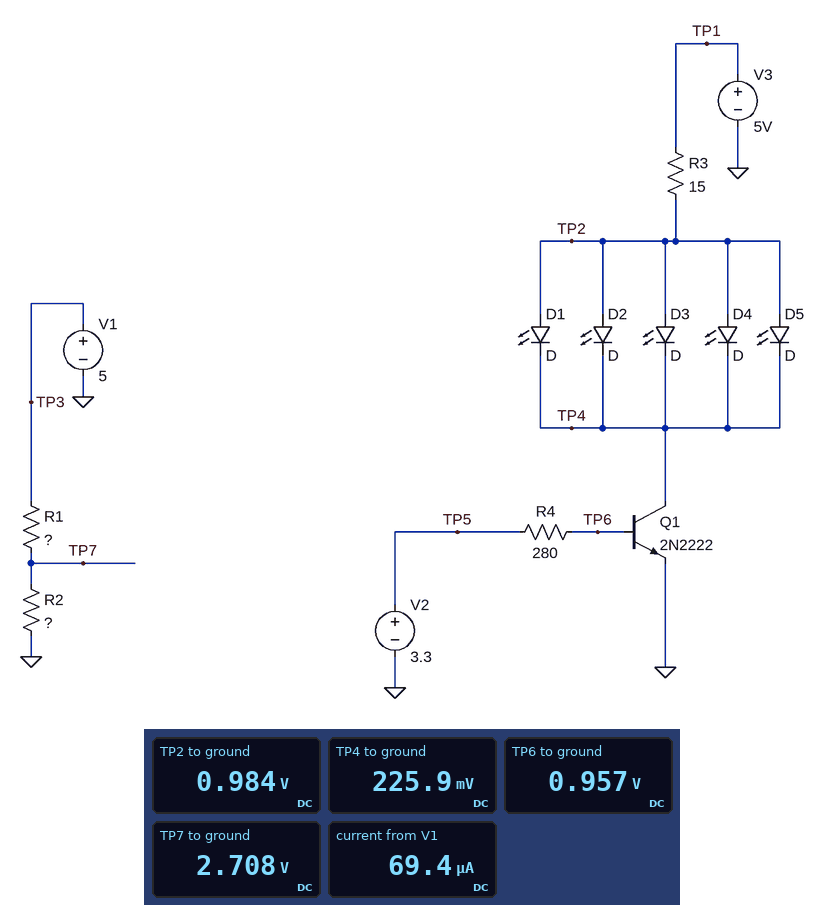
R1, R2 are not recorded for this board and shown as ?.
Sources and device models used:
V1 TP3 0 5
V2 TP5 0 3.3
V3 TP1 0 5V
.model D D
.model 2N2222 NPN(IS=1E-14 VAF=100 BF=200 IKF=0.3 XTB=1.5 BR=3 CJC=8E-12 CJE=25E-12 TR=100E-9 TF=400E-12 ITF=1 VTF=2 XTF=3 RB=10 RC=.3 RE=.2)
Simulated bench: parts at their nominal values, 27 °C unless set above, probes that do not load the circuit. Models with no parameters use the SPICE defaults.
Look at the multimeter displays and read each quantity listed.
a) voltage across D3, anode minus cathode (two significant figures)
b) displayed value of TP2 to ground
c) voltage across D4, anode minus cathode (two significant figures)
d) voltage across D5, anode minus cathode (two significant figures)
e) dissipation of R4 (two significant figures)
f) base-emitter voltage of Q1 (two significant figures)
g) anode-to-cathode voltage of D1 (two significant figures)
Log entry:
760 mV
0.984 V
760 mV
760 mV
20 mW
960 mV
760 mV
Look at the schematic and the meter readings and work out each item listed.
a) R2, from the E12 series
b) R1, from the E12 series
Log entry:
39 kΩ
33 kΩ
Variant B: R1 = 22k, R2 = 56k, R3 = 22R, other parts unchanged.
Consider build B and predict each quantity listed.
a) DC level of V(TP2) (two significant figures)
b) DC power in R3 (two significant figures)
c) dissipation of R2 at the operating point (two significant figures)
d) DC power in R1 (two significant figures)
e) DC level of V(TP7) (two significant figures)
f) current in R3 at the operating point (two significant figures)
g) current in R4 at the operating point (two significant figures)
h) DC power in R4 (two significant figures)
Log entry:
920 mV
760 mW
230 µW
90 µW
3.6 V
190 mA
8.5 mA
20 mW
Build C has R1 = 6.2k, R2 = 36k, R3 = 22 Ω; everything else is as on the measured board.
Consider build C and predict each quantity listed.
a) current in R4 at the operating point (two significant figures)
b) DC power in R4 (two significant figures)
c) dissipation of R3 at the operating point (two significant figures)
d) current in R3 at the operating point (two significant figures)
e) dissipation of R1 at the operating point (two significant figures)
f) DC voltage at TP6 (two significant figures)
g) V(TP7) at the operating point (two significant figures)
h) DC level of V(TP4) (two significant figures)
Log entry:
8.5 mA
20 mW
760 mW
190 mA
87 µW
930 mV
4.3 V
170 mV
